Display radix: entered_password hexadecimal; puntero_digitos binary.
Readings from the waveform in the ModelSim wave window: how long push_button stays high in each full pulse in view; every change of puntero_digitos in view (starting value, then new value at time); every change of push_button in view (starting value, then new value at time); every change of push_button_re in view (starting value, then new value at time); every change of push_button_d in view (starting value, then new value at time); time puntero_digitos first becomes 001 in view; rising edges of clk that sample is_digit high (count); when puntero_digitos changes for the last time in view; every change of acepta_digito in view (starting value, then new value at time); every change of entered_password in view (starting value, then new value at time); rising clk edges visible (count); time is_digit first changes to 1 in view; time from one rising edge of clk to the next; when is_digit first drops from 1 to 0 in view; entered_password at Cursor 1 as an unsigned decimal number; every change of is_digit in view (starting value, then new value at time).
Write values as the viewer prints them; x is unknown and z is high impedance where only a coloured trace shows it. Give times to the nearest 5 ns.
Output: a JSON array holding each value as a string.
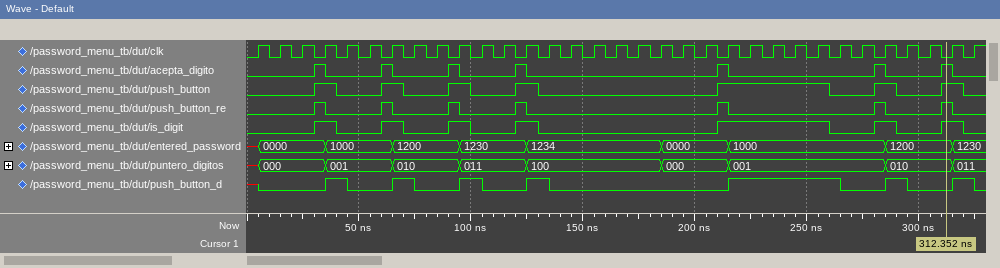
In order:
["10 ns, 10 ns, 10 ns, 10 ns, 50 ns, 10 ns, 10 ns", "x, 000 at 5 ns, 001 at 35 ns, 010 at 65 ns, 011 at 95 ns, 100 at 125 ns, 000 at 185 ns, 001 at 215 ns, 010 at 285 ns, 011 at 315 ns", "0, 1 at 30 ns, 0 at 40 ns, 1 at 60 ns, 0 at 70 ns, 1 at 90 ns, 0 at 100 ns, 1 at 120 ns, 0 at 130 ns, 1 at 210 ns, 0 at 260 ns, 1 at 280 ns, 0 at 290 ns, 1 at 310 ns, 0 at 320 ns", "0, 1 at 30 ns, 0 at 35 ns, 1 at 60 ns, 0 at 65 ns, 1 at 90 ns, 0 at 95 ns, 1 at 120 ns, 0 at 125 ns, 1 at 210 ns, 0 at 215 ns, 1 at 280 ns, 0 at 285 ns, 1 at 310 ns, 0 at 315 ns", "x, 0 at 5 ns, 1 at 35 ns, 0 at 45 ns, 1 at 65 ns, 0 at 75 ns, 1 at 95 ns, 0 at 105 ns, 1 at 125 ns, 0 at 135 ns, 1 at 215 ns, 0 at 265 ns, 1 at 285 ns, 0 at 295 ns, 1 at 315 ns, 0 at 325 ns", "35 ns", "11", "315 ns", "0, 1 at 30 ns, 0 at 35 ns, 1 at 60 ns, 0 at 65 ns, 1 at 90 ns, 0 at 95 ns, 1 at 120 ns, 0 at 125 ns, 1 at 210 ns, 0 at 215 ns, 1 at 280 ns, 0 at 285 ns, 1 at 310 ns, 0 at 315 ns", "x, 0000 at 5 ns, 1000 at 35 ns, 1200 at 65 ns, 1230 at 95 ns, 1234 at 125 ns, 0000 at 185 ns, 1000 at 215 ns, 1200 at 285 ns, 1230 at 315 ns", "33", "30 ns", "10 ns", "40 ns", "4608", "0, 1 at 30 ns, 0 at 40 ns, 1 at 60 ns, 0 at 70 ns, 1 at 90 ns, 0 at 100 ns, 1 at 120 ns, 0 at 130 ns, 1 at 210 ns, 0 at 260 ns, 1 at 280 ns, 0 at 290 ns, 1 at 310 ns, 0 at 320 ns"]
